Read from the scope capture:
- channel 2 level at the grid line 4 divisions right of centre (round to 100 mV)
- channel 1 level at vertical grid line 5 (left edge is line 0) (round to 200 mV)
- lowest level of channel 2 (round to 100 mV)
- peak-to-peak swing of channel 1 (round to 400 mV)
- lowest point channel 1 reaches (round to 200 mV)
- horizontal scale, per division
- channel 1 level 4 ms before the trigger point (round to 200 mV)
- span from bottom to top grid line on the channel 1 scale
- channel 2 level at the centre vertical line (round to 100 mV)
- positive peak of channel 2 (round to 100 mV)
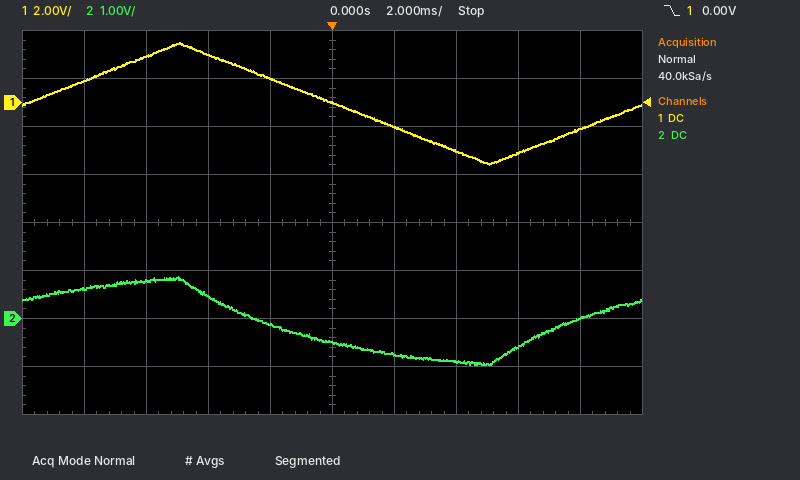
0.0 V
0.0 V
-1.0 V
5.2 V
-2.6 V
2 ms
2.0 V
16 V
-500 mV
900 mV
